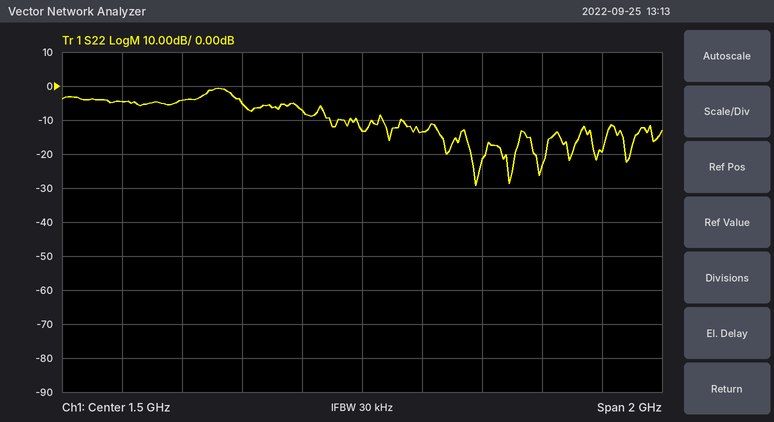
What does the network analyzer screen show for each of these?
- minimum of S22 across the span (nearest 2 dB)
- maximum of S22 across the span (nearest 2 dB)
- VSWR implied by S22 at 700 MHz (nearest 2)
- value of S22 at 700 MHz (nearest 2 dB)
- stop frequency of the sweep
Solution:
-30 dB
0 dB
4
-4 dB
2.5 GHz
